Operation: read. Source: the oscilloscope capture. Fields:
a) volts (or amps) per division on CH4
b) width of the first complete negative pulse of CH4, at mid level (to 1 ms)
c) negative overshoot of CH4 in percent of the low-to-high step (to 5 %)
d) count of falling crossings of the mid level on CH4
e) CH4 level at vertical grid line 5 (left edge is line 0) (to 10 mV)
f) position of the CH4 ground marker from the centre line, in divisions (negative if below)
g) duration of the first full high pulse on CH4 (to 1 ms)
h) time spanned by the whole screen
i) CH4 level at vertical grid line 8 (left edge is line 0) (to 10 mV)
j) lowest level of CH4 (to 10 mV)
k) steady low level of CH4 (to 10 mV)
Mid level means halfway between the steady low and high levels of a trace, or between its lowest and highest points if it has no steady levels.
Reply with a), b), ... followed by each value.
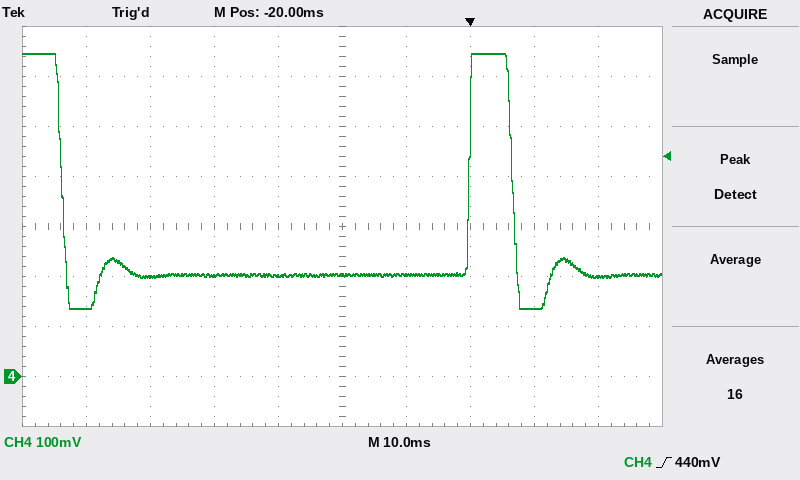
a) 100 mV
b) 64 ms
c) 15 %
d) 2
e) 200 mV
f) -3.0 div
g) 7 ms
h) 100 ms
i) 140 mV
j) 140 mV
k) 200 mV
